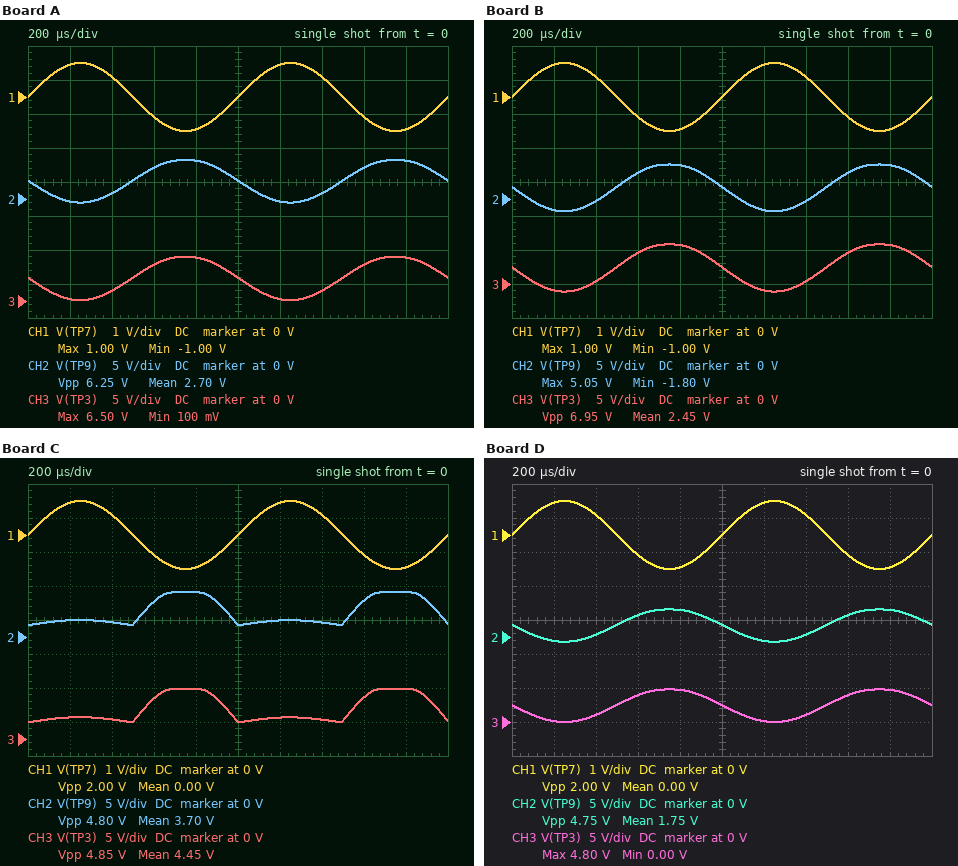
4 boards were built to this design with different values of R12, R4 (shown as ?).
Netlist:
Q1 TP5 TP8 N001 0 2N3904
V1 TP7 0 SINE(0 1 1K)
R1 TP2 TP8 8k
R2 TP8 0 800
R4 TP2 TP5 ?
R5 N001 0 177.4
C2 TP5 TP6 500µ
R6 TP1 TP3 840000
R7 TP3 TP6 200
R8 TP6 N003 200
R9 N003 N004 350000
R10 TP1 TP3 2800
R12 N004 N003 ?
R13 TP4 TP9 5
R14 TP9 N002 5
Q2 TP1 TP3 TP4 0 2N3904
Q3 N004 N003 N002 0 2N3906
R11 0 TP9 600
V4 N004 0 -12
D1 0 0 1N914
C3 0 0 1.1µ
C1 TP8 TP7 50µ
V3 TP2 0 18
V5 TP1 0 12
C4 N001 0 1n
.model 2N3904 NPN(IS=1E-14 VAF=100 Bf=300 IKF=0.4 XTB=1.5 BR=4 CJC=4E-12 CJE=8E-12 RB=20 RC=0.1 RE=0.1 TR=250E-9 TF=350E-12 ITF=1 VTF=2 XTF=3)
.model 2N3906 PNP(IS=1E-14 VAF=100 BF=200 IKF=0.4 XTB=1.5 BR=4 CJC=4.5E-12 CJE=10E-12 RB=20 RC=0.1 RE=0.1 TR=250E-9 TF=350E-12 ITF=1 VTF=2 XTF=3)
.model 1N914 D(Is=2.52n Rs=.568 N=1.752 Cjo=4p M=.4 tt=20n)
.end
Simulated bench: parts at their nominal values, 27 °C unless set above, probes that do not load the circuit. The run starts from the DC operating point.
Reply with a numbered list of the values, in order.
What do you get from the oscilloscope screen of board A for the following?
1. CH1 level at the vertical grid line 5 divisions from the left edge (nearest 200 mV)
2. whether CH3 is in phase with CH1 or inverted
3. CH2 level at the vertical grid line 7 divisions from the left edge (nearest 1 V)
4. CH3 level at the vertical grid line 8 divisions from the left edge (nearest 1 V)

1. 0 V
2. inverted
3. 1 V
4. 5 V
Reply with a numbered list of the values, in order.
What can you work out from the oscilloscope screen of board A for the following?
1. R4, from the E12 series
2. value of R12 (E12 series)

1. 1 kΩ
2. 4.7 kΩ
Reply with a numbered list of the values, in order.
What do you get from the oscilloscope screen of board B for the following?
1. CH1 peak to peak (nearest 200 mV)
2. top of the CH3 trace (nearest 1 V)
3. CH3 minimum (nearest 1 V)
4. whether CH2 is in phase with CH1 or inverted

1. 2.0 V
2. 6 V
3. -1 V
4. inverted
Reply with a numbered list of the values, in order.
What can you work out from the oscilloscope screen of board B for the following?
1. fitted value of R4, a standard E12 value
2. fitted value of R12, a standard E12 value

1. 1.2 kΩ
2. 3.9 kΩ
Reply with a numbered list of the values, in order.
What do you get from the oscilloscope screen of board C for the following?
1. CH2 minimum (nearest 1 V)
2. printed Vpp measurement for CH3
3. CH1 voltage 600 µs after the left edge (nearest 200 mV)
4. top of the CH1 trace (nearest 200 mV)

1. 2 V
2. 4.85 V
3. -600 mV
4. 1.0 V
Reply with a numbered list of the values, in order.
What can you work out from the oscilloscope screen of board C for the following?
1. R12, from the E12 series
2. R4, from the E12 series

1. 3.9 kΩ
2. 3.9 kΩ
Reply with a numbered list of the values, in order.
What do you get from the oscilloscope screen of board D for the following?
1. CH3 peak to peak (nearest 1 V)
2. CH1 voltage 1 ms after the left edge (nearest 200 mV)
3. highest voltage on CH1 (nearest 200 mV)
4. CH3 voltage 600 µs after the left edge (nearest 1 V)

1. 5 V
2. 0 V
3. 1.0 V
4. 4 V
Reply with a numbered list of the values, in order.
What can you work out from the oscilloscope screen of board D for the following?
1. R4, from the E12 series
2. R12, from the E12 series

1. 680 Ω
2. 3.9 kΩ
